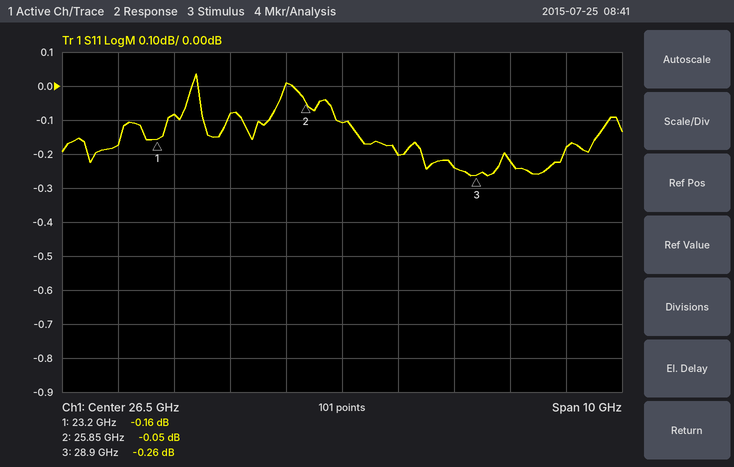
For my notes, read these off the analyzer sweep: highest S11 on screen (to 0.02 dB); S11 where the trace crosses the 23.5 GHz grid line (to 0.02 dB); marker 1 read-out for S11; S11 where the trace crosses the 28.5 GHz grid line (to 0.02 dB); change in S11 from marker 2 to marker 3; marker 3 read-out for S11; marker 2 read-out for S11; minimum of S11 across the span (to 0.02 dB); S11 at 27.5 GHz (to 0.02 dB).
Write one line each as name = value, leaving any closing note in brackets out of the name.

highest S11 on screen = 0.04 dB
S11 where the trace crosses the 23.5 GHz grid line = -0.08 dB
marker 1 read-out for S11 = -0.16 dB
S11 where the trace crosses the 28.5 GHz grid line = -0.24 dB
change in S11 from marker 2 to marker 3 = -0.21 dB
marker 3 read-out for S11 = -0.26 dB
marker 2 read-out for S11 = -0.05 dB
minimum of S11 across the span = -0.26 dB
S11 at 27.5 GHz = -0.20 dB
